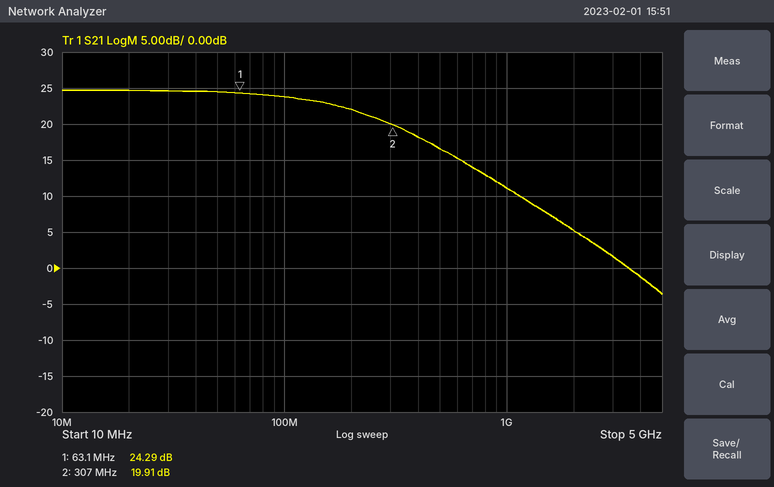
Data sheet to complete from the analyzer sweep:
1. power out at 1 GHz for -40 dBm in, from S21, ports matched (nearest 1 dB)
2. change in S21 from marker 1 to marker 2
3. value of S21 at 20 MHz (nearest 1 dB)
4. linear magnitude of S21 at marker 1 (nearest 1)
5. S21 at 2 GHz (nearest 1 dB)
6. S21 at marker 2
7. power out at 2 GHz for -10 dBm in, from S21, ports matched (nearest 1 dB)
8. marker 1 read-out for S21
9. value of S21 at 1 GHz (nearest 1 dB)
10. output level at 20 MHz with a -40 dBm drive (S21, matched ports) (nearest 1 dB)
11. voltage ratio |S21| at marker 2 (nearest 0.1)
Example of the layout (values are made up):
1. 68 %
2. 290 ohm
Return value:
1. -29 dBm
2. -4.38 dB
3. 25 dB
4. 16
5. 5 dB
6. 19.91 dB
7. -5 dBm
8. 24.29 dB
9. 11 dB
10. -15 dBm
11. 9.9
